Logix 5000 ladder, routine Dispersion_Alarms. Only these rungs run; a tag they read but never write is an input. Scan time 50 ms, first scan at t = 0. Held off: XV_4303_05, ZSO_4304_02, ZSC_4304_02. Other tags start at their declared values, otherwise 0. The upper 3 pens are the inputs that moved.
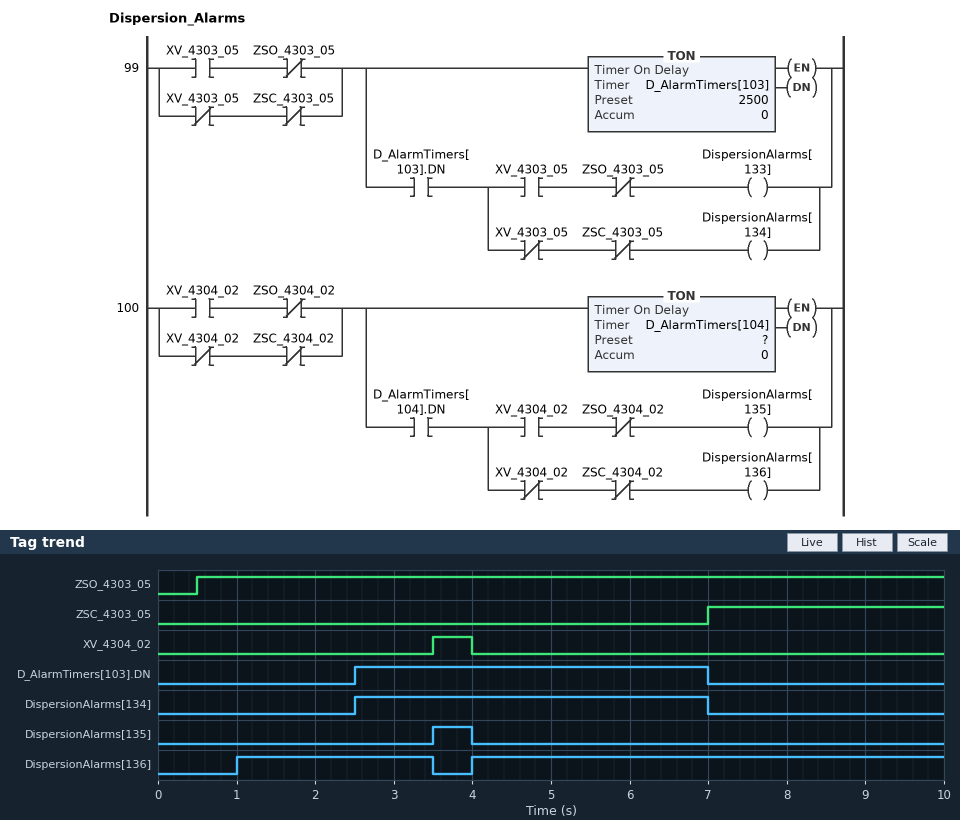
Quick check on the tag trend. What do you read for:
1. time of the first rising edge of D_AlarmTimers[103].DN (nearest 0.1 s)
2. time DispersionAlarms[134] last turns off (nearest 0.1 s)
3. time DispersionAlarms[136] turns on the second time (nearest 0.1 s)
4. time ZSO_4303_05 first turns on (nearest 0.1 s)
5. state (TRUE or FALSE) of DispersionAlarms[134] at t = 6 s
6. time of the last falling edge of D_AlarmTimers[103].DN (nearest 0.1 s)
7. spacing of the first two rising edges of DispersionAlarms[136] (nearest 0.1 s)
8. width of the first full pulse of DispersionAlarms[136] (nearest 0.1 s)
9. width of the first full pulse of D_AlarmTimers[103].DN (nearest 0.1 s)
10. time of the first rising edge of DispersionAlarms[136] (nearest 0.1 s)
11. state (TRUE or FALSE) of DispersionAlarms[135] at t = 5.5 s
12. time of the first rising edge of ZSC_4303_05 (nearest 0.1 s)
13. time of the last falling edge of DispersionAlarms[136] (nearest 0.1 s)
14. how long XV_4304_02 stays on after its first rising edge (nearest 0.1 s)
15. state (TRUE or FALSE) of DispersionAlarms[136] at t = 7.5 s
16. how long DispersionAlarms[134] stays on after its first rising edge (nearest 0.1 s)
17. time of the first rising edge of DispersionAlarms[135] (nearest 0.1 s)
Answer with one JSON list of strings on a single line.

["2.5 s", "7.0 s", "4.0 s", "0.5 s", "TRUE", "7.0 s", "3.0 s", "2.5 s", "4.5 s", "1.0 s", "FALSE", "7.0 s", "3.5 s", "0.5 s", "TRUE", "4.5 s", "3.5 s"]
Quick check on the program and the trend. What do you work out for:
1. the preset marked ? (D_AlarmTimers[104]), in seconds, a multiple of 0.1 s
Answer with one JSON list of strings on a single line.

["1.0 s"]
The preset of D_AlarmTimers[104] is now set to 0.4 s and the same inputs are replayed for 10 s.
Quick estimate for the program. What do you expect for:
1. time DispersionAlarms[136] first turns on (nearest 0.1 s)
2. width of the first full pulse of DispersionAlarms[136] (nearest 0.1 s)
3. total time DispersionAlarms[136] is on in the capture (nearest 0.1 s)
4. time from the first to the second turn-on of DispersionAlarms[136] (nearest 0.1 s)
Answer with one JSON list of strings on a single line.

["0.4 s", "3.1 s", "9.1 s", "3.6 s"]
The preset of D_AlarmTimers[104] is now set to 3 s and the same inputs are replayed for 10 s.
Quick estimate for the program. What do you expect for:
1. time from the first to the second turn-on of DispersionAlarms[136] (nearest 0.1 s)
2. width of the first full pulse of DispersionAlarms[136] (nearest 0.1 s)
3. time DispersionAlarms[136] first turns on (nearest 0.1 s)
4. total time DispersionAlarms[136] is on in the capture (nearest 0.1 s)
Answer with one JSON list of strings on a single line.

["1.0 s", "0.5 s", "3.0 s", "6.5 s"]
